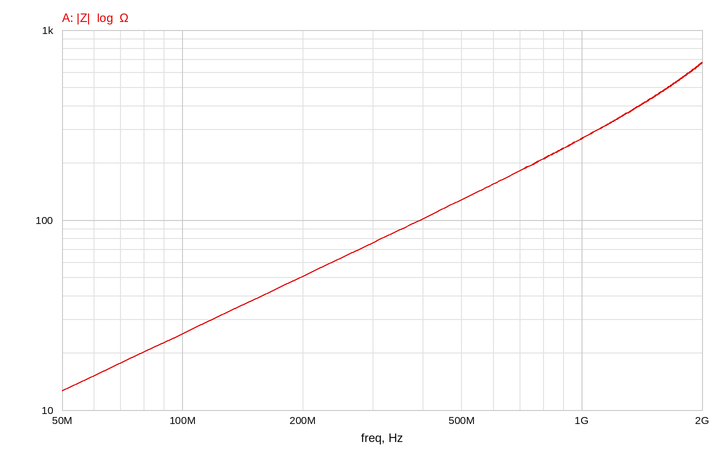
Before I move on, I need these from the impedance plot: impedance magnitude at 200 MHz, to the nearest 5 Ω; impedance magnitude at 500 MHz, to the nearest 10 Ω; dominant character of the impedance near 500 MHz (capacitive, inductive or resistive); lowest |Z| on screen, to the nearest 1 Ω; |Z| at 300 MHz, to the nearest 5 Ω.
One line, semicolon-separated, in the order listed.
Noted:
50 Ω; 130 Ω; inductive; 13 Ω; 75 Ω
